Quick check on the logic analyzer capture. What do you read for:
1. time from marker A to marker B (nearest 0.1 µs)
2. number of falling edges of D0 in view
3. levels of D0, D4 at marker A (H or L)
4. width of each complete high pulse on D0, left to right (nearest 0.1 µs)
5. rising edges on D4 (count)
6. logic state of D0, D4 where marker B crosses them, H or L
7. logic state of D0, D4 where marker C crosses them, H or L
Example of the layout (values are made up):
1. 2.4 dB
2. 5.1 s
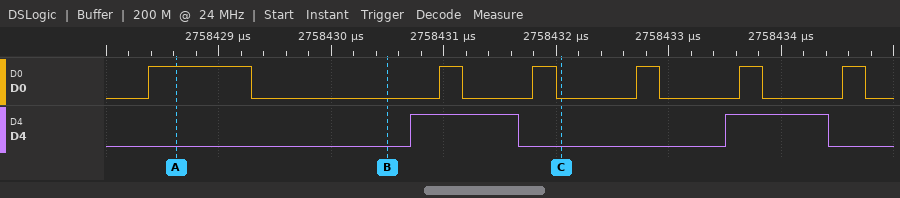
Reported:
1. 1.9 µs
2. 6
3. D0=H, D4=L
4. 0.9 µs, 0.2 µs, 0.2 µs, 0.2 µs, 0.2 µs, 0.2 µs
5. 2
6. D0=L, D4=L
7. D0=L, D4=L
